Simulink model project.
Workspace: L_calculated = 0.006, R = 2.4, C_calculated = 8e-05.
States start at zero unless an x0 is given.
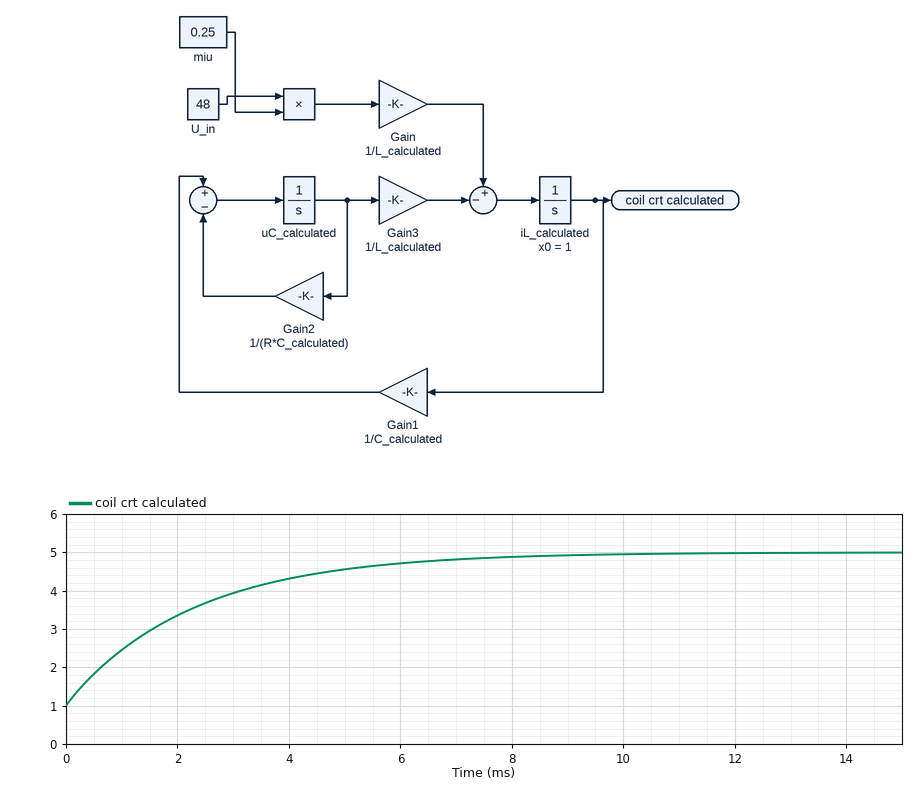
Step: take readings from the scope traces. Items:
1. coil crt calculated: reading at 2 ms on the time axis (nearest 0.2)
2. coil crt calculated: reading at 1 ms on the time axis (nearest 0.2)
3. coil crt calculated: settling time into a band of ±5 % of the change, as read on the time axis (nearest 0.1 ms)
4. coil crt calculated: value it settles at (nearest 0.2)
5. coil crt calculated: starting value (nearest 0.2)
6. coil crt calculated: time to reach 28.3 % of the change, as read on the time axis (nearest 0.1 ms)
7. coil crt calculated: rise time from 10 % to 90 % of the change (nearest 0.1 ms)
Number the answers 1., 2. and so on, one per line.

1. 3.4
2. 2.4
3. 6.8 ms
4. 5.0
5. 1.0
6. 0.7 ms
7. 5.0 ms
